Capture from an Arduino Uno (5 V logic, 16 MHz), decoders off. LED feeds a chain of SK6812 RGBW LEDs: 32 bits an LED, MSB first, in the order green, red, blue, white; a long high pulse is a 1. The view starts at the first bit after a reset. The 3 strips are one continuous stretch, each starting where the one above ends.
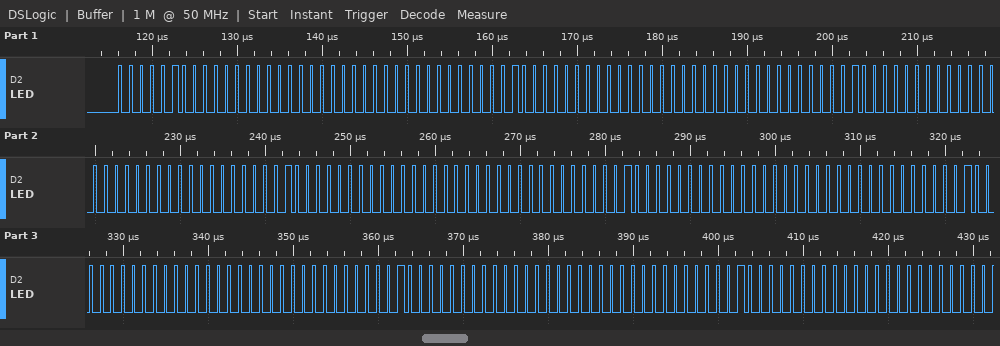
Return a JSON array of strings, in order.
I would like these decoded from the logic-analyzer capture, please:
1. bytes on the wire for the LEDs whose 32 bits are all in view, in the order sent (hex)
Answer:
["04 00 00 00 04 00 00 00 04 00 00 00 04 00 00 00 04 00 00 00 04 00 00 00 04 00 00 00"]
